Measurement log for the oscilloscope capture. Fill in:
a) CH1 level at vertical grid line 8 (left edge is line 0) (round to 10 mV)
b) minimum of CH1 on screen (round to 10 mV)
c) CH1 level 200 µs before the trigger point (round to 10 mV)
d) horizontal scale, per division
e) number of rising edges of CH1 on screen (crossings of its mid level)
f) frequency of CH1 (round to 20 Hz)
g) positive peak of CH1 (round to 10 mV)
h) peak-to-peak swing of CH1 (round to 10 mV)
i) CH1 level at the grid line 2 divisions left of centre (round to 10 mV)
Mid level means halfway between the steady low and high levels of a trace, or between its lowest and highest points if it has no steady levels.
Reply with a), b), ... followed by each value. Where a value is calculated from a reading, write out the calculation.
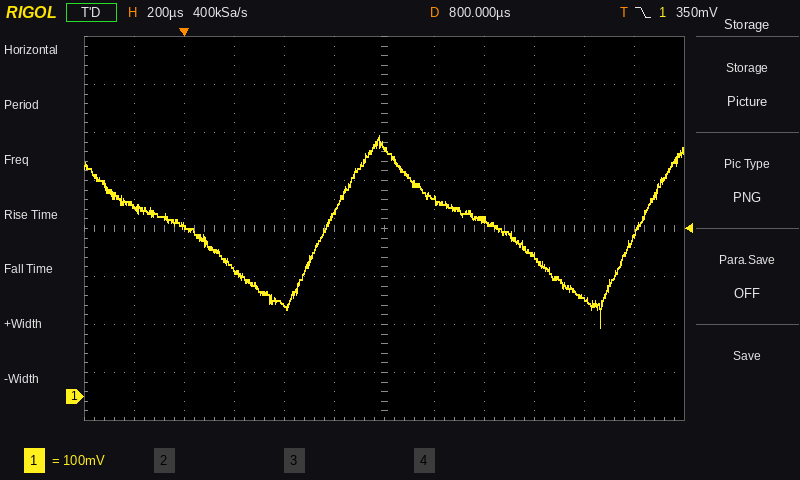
a) 370 mV
b) 140 mV
c) 400 mV
d) 200 µs
e) 2
f) 800 Hz
g) 540 mV
h) 540 mV − (140 mV) = 400 mV
i) 190 mV
